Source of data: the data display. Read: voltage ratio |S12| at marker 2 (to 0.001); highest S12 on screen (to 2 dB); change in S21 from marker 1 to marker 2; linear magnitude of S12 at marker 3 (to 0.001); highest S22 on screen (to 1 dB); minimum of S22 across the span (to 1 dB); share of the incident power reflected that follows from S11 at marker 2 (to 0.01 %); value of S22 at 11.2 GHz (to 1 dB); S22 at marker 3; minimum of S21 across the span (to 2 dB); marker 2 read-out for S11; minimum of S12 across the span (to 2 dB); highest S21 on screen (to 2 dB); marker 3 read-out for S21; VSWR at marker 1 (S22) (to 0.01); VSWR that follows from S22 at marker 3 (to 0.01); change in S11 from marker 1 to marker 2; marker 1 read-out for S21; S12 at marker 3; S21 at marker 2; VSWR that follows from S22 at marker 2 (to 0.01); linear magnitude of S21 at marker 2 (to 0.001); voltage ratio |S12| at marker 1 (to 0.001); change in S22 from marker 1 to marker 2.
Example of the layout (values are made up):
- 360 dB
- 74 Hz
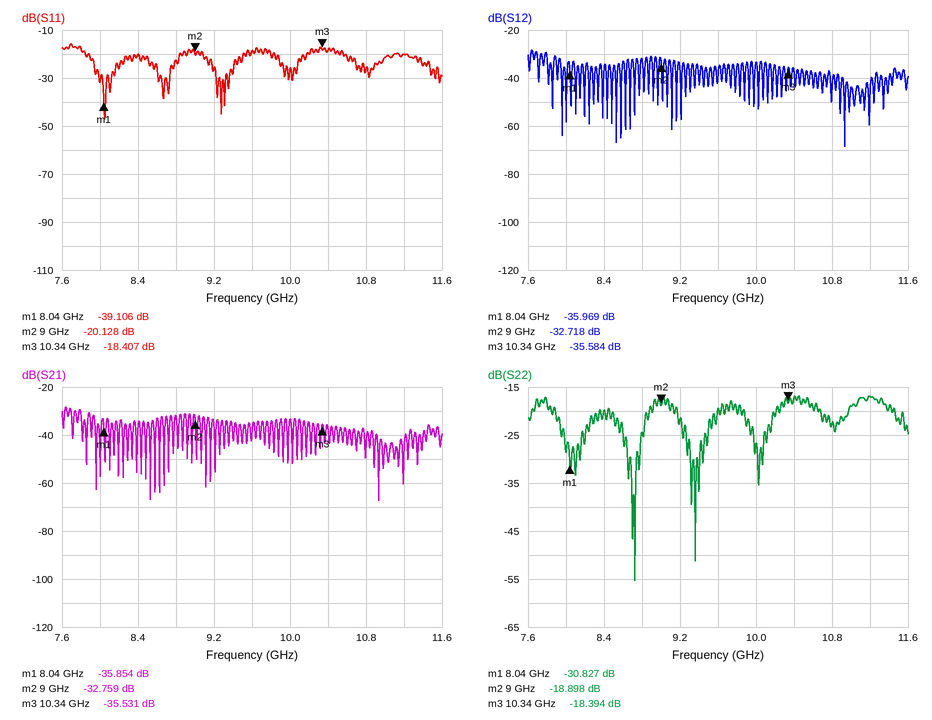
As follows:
- 0.023
- -28 dB
- 3.095 dB
- 0.017
- -17 dB
- -55 dB
- 0.97 %
- -17 dB
- -18.394 dB
- -68 dB
- -20.128 dB
- -68 dB
- -28 dB
- -35.531 dB
- 1.06
- 1.27
- 18.978 dB
- -35.854 dB
- -35.584 dB
- -32.759 dB
- 1.26
- 0.023
- 0.016
- 11.929 dB
